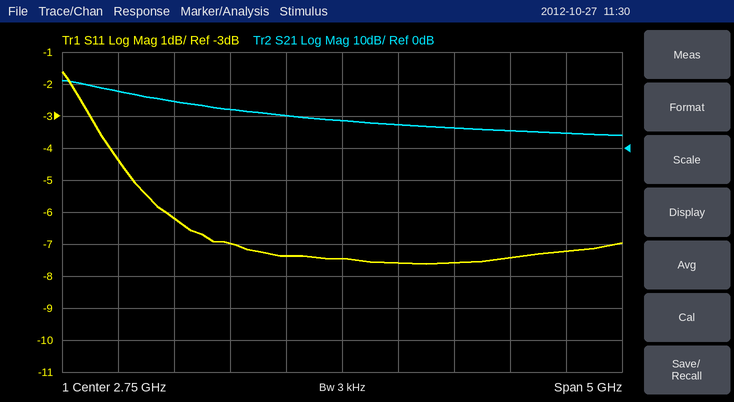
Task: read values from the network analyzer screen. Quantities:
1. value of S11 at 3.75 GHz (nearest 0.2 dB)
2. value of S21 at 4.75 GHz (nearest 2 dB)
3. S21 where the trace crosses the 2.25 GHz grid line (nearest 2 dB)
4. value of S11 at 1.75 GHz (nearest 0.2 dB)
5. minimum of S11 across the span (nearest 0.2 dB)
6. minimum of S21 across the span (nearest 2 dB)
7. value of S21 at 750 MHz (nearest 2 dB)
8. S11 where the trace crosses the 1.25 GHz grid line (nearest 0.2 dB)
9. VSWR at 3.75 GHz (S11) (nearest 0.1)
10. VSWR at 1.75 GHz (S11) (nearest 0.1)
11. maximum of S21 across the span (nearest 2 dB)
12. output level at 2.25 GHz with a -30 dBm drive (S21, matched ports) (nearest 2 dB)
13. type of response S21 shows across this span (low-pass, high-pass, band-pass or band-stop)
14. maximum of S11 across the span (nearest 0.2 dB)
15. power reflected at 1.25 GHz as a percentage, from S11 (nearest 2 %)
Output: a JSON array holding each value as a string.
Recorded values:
["-7.6 dB", "4 dB", "10 dB", "-7.0 dB", "-7.6 dB", "4 dB", "18 dB", "-6.2 dB", "2.4", "2.6", "22 dB", "-20 dBm", "low-pass", "-1.6 dB", "24 %"]
